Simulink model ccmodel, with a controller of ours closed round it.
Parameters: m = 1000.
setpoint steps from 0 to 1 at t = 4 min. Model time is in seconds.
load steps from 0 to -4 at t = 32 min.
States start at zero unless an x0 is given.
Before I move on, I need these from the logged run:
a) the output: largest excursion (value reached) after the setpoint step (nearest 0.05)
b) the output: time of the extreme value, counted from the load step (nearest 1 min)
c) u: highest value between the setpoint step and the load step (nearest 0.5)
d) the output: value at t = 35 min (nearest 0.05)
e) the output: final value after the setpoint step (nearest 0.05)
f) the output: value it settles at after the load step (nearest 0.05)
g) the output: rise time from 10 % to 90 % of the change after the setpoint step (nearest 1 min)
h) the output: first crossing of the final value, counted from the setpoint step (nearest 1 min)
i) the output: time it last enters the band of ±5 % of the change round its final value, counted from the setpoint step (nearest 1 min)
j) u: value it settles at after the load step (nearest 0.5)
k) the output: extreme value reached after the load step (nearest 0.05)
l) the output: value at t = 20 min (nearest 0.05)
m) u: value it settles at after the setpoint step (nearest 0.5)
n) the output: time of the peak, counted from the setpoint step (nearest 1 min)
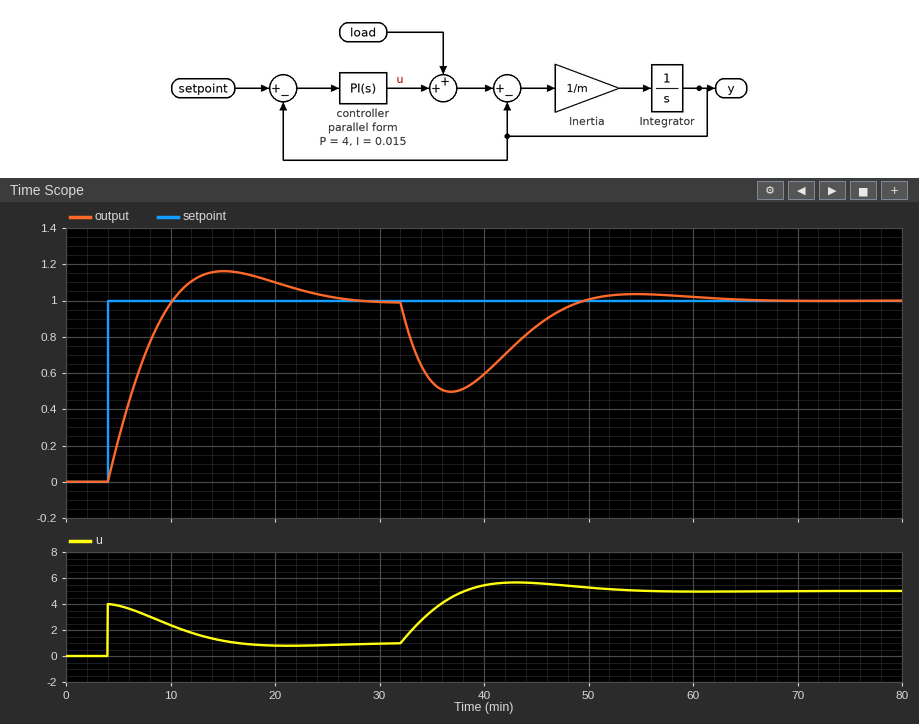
1.15
5 min
4.0
0.55
1.00
1.00
5 min
6 min
19 min
5.0
0.50
1.10
1.0
11 min
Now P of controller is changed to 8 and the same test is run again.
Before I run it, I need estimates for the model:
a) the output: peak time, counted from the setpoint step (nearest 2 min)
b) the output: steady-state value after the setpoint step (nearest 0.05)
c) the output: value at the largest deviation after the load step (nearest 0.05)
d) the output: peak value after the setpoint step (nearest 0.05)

10 min
1.00
0.65
1.05
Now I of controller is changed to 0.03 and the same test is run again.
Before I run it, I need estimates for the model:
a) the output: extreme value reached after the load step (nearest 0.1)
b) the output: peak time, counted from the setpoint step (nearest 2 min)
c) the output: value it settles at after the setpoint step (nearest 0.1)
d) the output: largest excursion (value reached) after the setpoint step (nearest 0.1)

0.6
8 min
1.0
1.3
